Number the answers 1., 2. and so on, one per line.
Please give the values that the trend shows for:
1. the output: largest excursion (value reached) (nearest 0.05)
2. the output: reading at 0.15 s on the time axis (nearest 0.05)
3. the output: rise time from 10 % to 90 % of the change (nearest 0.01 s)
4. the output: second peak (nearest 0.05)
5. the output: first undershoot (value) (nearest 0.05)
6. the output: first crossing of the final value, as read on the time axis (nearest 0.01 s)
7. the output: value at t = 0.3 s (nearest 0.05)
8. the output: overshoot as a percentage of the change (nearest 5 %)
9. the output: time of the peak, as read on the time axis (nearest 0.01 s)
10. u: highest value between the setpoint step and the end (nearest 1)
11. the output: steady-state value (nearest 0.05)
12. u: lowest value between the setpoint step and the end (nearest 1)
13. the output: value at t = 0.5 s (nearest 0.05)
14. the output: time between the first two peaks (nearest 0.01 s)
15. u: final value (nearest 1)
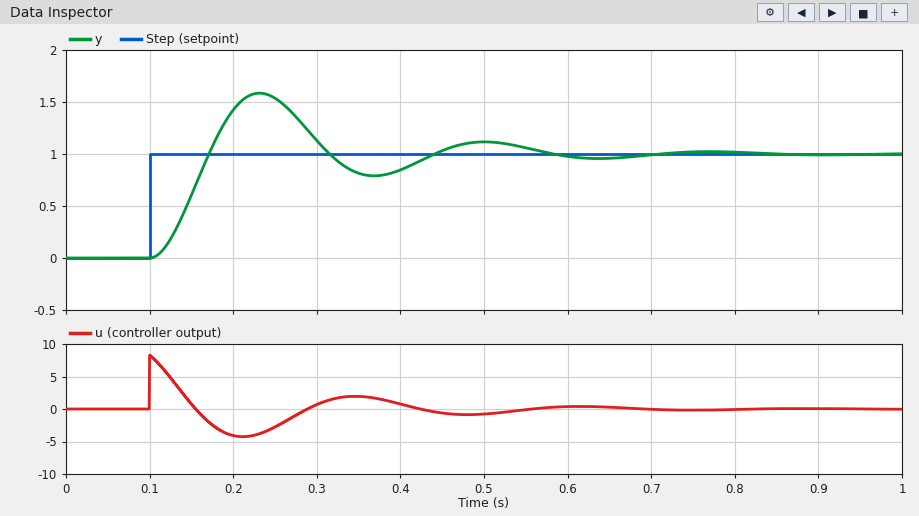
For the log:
1. 1.60
2. 0.60
3. 0.05 s
4. 1.10
5. 0.80
6. 0.17 s
7. 1.15
8. 60 %
9. 0.23 s
10. 8
11. 1.00
12. -4
13. 1.10
14. 0.27 s
15. 0
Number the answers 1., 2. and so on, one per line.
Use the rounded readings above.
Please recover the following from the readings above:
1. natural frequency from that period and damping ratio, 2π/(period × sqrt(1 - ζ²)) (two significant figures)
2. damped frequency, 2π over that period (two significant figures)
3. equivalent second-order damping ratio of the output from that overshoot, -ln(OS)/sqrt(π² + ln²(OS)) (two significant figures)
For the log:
1. 24 rad/s
2. 23 rad/s
3. 0.16
